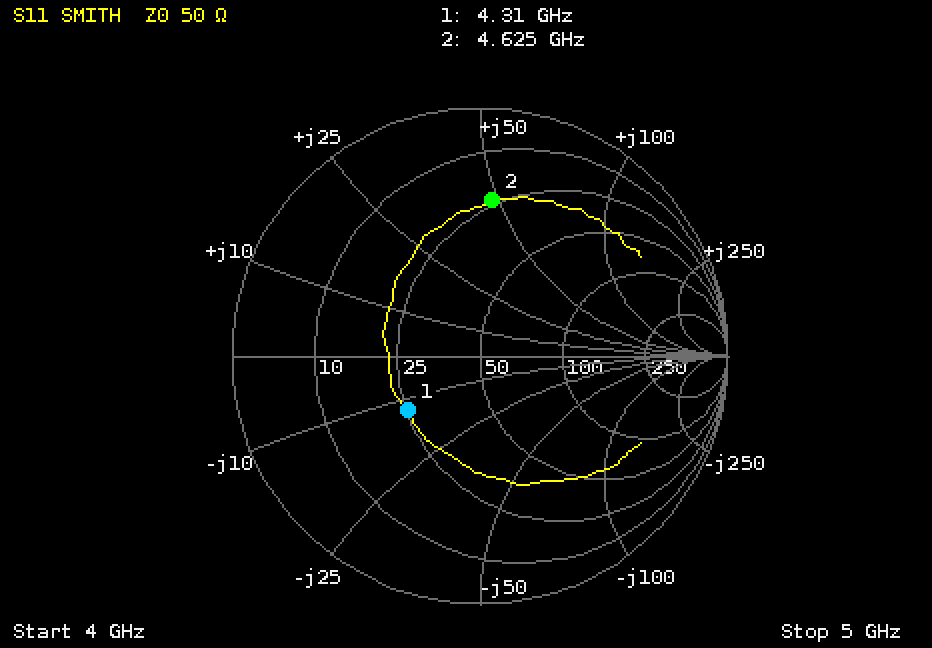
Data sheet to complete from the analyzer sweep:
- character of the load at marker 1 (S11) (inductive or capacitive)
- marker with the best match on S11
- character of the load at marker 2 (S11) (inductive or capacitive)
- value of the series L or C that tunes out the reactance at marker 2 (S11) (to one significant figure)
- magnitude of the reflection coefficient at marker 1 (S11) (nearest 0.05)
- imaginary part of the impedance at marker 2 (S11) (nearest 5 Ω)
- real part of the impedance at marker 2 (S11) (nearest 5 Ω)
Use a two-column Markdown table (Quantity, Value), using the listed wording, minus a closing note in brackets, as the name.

| Quantity | Value |
|---|---|
| character of the load at marker 1 (S11) | capacitive |
| marker with the best match on S11 | marker 1 |
| character of the load at marker 2 (S11) | inductive |
| value of the series L or C that tunes out the reactance at marker 2 (S11) | 700 fF |
| magnitude of the reflection coefficient at marker 1 (S11) | 0.35 |
| imaginary part of the impedance at marker 2 (S11) | +50 Ω |
| real part of the impedance at marker 2 (S11) | 25 Ω |
